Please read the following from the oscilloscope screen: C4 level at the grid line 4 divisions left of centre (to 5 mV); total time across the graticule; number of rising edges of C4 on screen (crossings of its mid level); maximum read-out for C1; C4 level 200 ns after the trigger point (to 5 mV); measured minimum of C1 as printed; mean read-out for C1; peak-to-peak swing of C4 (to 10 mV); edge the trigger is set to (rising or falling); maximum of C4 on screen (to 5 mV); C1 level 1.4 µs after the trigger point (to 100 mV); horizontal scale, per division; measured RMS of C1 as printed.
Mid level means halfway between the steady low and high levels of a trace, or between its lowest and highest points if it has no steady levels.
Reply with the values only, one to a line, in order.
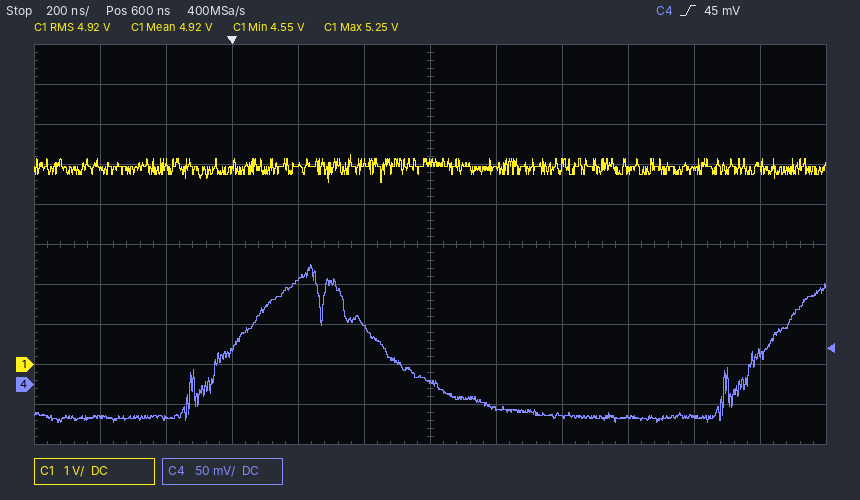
-40 mV
2.4 µs
2
5.25 V
130 mV
4.55 V
4.92 V
200 mV
rising
150 mV
4.9 V
200 ns
4.92 V
